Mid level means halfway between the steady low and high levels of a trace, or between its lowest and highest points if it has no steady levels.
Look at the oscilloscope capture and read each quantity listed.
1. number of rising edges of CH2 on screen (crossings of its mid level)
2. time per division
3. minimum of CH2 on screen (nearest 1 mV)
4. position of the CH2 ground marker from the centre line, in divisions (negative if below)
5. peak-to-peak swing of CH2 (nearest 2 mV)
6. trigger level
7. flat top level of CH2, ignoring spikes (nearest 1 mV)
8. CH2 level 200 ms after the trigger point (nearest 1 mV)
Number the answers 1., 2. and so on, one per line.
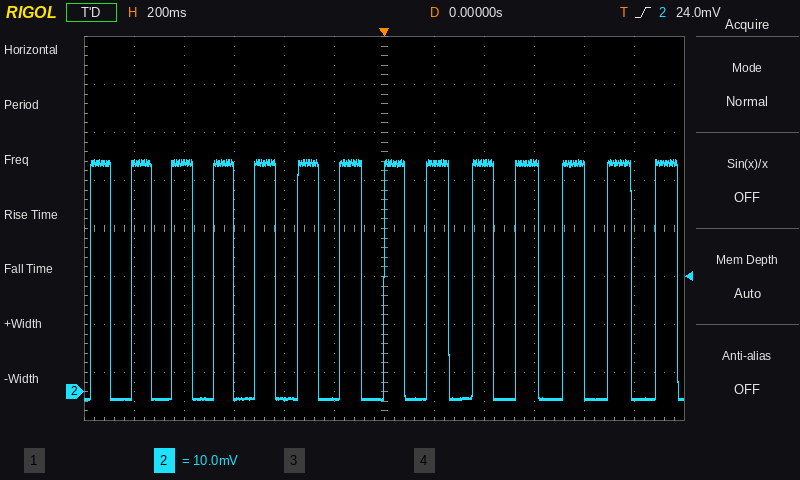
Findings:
1. 14
2. 200 ms
3. -2 mV
4. -3.4 div
5. 50 mV
6. 24.0 mV
7. 48 mV
8. 48 mV
